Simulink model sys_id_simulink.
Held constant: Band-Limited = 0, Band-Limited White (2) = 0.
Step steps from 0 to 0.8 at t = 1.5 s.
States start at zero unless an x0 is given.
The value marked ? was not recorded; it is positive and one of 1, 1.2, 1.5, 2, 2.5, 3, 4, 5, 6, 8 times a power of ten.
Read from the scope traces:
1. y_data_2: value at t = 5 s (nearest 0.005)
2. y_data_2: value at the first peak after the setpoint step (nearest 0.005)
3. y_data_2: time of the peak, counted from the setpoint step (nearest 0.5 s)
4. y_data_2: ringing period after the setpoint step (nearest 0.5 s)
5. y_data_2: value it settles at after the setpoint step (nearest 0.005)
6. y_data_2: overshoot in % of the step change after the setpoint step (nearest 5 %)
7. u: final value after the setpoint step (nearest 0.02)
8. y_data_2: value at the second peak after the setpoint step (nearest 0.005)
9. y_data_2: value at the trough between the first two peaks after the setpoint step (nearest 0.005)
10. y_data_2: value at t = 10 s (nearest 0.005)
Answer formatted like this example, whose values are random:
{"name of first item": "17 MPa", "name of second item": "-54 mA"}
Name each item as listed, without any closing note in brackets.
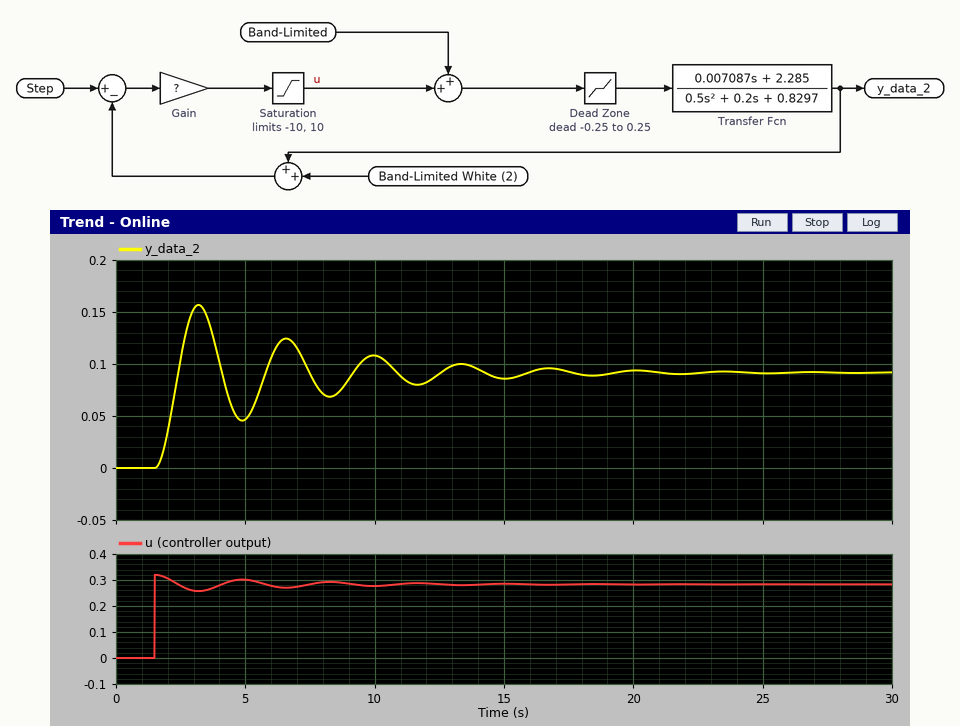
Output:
{"y_data_2: value at t = 5 s": "0.045", "y_data_2: value at the first peak after the setpoint step": "0.155", "y_data_2: time of the peak, counted from the setpoint step": "1.5 s", "y_data_2: ringing period after the setpoint step": "3.5 s", "y_data_2: value it settles at after the setpoint step": "0.090", "y_data_2: overshoot in % of the step change after the setpoint step": "70 %", "u: final value after the setpoint step": "0.28", "y_data_2: value at the second peak after the setpoint step": "0.125", "y_data_2: value at the trough between the first two peaks after the setpoint step": "0.045", "y_data_2: value at t = 10 s": "0.110"}
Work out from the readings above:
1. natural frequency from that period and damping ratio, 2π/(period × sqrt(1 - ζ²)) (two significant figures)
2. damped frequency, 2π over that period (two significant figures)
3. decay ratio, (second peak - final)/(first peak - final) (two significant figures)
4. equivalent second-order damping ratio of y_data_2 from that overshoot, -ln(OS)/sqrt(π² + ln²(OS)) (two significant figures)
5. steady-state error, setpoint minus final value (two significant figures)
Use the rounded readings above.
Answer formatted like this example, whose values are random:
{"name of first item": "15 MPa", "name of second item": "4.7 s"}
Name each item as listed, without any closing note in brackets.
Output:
{"natural frequency from that period and damping ratio, 2π/(period × sqrt(1 - ζ²))": "1.8 rad/s", "damped frequency, 2π over that period": "1.8 rad/s", "decay ratio, (second peak - final)/(first peak - final)": "0.54", "equivalent second-order damping ratio of y_data_2 from that overshoot, -ln(OS)/sqrt(π² + ln²(OS))": "0.11", "steady-state error, setpoint minus final value": "0.71"}
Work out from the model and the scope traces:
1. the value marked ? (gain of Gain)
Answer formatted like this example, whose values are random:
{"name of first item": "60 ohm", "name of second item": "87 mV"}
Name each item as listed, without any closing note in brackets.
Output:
{"the value marked ?": "0.4"}
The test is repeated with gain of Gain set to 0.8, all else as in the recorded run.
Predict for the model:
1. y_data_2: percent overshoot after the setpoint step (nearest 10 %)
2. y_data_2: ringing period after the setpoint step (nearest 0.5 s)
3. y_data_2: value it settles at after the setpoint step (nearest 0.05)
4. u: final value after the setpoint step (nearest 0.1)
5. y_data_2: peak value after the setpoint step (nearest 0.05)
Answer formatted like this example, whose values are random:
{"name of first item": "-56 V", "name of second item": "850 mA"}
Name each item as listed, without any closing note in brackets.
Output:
{"y_data_2: percent overshoot after the setpoint step": "80 %", "y_data_2: ringing period after the setpoint step": "3.0 s", "y_data_2: value it settles at after the setpoint step": "0.35", "u: final value after the setpoint step": "0.4", "y_data_2: peak value after the setpoint step": "0.60"}
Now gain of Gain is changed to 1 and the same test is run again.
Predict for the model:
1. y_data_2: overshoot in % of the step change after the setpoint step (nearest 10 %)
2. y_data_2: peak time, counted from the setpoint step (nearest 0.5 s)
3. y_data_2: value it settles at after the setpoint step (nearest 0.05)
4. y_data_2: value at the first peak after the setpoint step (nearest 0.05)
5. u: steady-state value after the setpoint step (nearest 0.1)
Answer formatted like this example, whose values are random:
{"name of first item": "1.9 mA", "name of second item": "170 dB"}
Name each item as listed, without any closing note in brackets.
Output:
{"y_data_2: overshoot in % of the step change after the setpoint step": "90 %", "y_data_2: peak time, counted from the setpoint step": "1.5 s", "y_data_2: value it settles at after the setpoint step": "0.40", "y_data_2: value at the first peak after the setpoint step": "0.75", "u: steady-state value after the setpoint step": "0.4"}
